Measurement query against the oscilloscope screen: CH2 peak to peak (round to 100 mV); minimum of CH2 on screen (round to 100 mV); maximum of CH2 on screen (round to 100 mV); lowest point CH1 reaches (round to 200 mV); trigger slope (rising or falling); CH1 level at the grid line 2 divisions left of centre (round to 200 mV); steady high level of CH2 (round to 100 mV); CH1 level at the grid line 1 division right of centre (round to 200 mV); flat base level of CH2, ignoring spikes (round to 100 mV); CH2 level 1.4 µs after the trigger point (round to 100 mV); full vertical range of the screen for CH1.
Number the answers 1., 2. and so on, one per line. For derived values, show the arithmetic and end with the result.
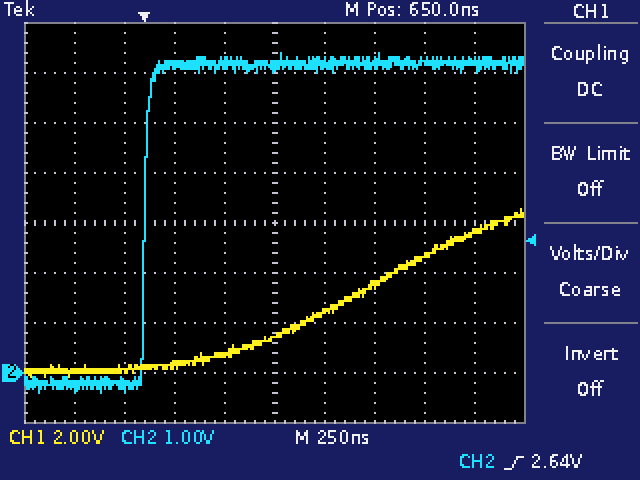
1. 6.4 V − (-400 mV) = 6.8 V
2. -400 mV
3. 6.4 V
4. -200 mV
5. rising
6. 400 mV
7. 6.2 V
8. 2.4 V
9. -200 mV
10. 6.2 V
11. 16 V
